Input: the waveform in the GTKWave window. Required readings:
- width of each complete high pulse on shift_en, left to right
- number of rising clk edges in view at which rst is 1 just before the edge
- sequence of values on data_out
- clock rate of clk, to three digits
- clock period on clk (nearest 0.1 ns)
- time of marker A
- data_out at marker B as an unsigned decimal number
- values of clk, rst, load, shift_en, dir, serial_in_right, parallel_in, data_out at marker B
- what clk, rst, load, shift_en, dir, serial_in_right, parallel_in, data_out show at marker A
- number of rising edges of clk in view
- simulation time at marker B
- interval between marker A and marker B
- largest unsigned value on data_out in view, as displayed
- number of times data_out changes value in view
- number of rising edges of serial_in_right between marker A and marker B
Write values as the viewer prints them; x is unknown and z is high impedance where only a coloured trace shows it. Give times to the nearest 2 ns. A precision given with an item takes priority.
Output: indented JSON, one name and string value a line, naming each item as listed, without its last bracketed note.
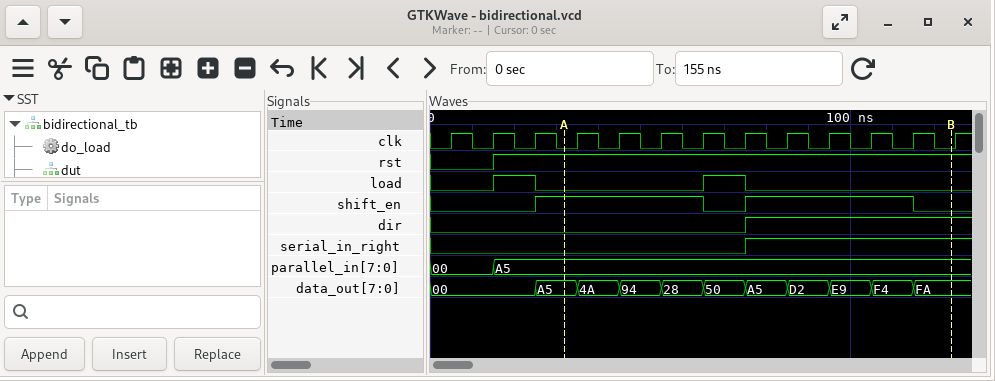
{
  "width of each complete high pulse on shift_en, left to right": "40 ns, 40 ns",
  "number of rising clk edges in view at which rst is 1 just before the edge": "11",
  "sequence of values on data_out": "00, A5, 4A, 94, 28, 50, A5, D2, E9, F4, FA",
  "clock rate of clk, to three digits": "100 MHz",
  "clock period on clk": "10 ns",
  "time of marker A": "32 ns",
  "data_out at marker B as an unsigned decimal number": "250",
  "values of clk, rst, load, shift_en, dir, serial_in_right, parallel_in, data_out at marker B": "clk=0, rst=1, load=0, shift_en=0, dir=1, serial_in_right=1, parallel_in=A5, data_out=FA",
  "what clk, rst, load, shift_en, dir, serial_in_right, parallel_in, data_out show at marker A": "clk=0, rst=1, load=0, shift_en=1, dir=0, serial_in_right=0, parallel_in=A5, data_out=A5",
  "number of rising edges of clk in view": "13",
  "simulation time at marker B": "124 ns",
  "interval between marker A and marker B": "92 ns",
  "largest unsigned value on data_out in view, as displayed": "FA",
  "number of times data_out changes value in view": "10",
  "number of rising edges of serial_in_right between marker A and marker B": "1"
}
